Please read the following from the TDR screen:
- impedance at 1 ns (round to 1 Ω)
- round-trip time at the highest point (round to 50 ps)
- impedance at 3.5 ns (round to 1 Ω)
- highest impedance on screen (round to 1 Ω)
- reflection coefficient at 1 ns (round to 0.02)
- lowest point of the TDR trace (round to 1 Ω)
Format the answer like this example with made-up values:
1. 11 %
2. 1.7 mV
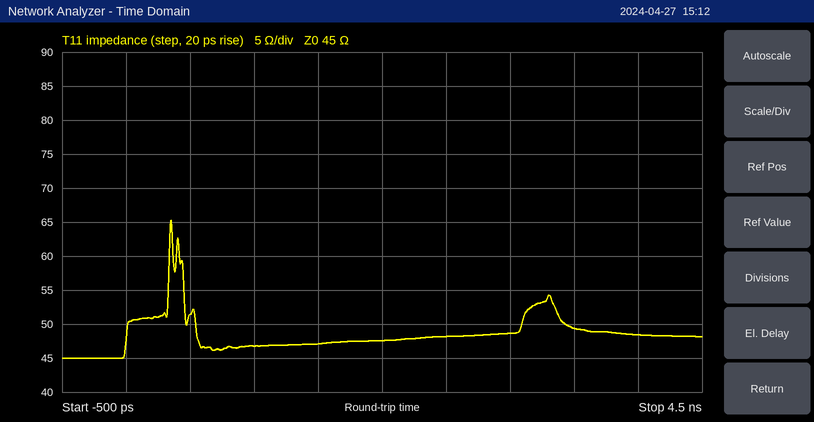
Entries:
1. 47 Ω
2. 350 ps
3. 49 Ω
4. 65 Ω
5. +0.02
6. 45 Ω
